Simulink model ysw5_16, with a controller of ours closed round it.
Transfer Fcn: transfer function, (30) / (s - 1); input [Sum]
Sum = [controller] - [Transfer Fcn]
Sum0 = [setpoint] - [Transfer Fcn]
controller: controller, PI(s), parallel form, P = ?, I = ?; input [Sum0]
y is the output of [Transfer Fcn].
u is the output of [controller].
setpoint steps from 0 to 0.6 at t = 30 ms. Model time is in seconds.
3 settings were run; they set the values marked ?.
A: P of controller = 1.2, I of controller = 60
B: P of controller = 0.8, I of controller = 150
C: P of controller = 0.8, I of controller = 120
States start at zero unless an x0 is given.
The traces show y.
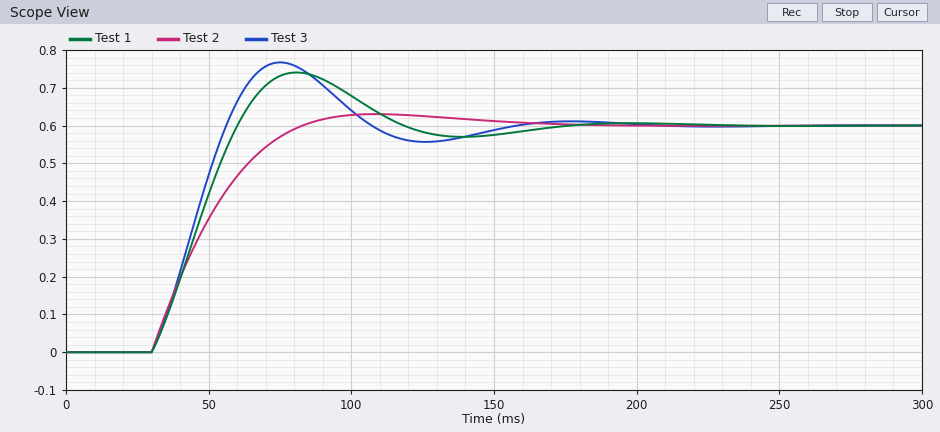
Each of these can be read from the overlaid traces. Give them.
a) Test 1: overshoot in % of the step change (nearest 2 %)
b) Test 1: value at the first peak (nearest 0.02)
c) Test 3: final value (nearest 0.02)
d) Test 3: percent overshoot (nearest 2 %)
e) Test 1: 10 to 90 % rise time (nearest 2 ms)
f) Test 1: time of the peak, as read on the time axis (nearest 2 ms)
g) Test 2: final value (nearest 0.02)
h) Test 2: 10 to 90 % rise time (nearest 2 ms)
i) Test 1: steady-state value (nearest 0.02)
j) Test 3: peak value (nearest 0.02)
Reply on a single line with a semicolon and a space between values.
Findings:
24 %; 0.74; 0.60; 28 %; 22 ms; 80 ms; 0.60; 36 ms; 0.60; 0.76
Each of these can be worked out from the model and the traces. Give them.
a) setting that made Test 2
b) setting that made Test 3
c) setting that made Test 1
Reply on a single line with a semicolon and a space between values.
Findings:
A; B; C
